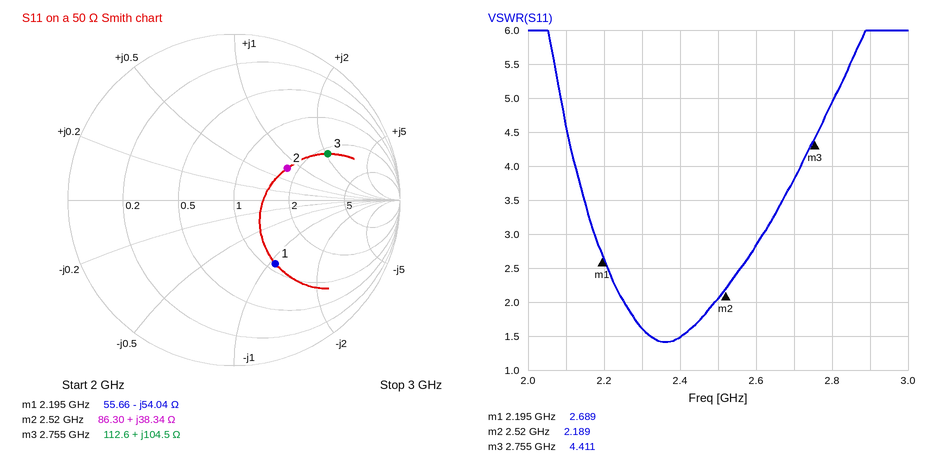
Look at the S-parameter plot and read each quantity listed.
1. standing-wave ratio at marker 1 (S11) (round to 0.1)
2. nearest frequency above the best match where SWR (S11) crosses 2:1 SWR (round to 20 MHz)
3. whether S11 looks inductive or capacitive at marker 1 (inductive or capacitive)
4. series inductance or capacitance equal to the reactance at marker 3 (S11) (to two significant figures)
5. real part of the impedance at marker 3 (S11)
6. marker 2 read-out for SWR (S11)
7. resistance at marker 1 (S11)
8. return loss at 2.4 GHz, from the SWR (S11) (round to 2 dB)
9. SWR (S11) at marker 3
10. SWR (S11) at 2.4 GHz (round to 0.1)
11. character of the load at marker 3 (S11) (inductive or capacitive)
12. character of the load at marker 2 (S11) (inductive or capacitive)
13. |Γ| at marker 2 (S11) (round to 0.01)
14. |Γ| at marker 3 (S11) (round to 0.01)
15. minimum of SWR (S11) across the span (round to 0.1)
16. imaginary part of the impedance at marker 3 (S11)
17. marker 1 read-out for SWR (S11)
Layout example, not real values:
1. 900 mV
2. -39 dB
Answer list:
1. 2.7
2. 2.50 GHz
3. capacitive
4. 6.0 nH
5. 112.6 Ω
6. 2.189
7. 55.66 Ω
8. 14 dB
9. 4.411
10. 1.5
11. inductive
12. inductive
13. 0.37
14. 0.63
15. 1.4
16. +104.5 Ω
17. 2.689
